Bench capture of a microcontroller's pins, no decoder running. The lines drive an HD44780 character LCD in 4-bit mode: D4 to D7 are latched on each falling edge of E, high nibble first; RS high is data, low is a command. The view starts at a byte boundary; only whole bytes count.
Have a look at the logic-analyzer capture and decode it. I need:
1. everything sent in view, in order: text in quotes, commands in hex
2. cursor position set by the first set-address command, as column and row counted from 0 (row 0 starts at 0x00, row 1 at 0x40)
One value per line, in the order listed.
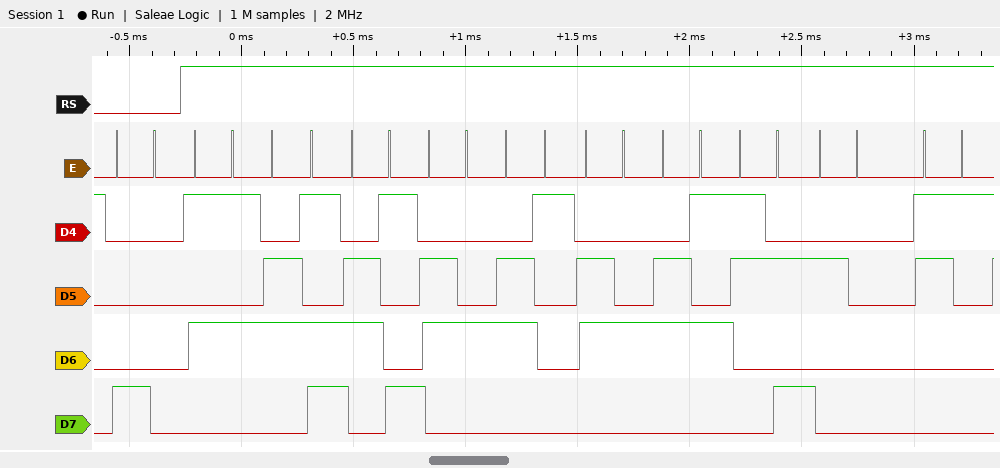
0x80 "Umidade: 1"
column 0, row 0
